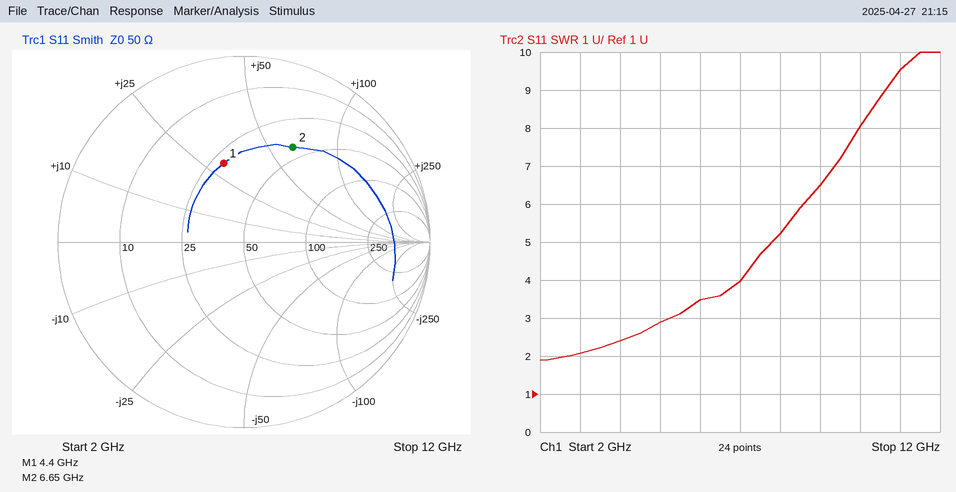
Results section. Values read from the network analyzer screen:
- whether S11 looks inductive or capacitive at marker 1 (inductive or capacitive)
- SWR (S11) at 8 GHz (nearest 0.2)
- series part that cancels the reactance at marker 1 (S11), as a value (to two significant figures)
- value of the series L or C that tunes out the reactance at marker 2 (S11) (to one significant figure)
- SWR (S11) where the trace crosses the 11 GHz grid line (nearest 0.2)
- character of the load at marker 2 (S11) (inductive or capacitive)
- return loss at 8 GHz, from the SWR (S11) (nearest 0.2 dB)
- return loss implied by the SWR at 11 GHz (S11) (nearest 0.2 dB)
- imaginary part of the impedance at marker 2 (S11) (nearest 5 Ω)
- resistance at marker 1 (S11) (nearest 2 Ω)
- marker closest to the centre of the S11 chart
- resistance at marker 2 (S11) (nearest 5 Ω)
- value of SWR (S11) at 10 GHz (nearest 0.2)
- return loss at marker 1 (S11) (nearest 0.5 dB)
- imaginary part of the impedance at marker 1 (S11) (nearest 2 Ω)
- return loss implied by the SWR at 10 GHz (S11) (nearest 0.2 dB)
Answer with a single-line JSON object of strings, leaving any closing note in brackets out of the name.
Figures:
{"whether S11 looks inductive or capacitive at marker 1": "inductive", "SWR (S11) at 8 GHz": "5.2", "series part that cancels the reactance at marker 1 (S11), as a value": "1.2 pF", "value of the series L or C that tunes out the reactance at marker 2 (S11)": "400 fF", "SWR (S11) where the trace crosses the 11 GHz grid line": "9.6", "character of the load at marker 2 (S11)": "inductive", "return loss at 8 GHz, from the SWR (S11)": "3.4 dB", "return loss implied by the SWR at 11 GHz (S11)": "1.8 dB", "imaginary part of the impedance at marker 2 (S11)": "+65 Ω", "resistance at marker 1 (S11)": "28 Ω", "marker closest to the centre of the S11 chart": "marker 1", "resistance at marker 2 (S11)": "40 Ω", "value of SWR (S11) at 10 GHz": "8.0", "return loss at marker 1 (S11)": "7.0 dB", "imaginary part of the impedance at marker 1 (S11)": "+30 Ω", "return loss implied by the SWR at 10 GHz (S11)": "2.2 dB"}
